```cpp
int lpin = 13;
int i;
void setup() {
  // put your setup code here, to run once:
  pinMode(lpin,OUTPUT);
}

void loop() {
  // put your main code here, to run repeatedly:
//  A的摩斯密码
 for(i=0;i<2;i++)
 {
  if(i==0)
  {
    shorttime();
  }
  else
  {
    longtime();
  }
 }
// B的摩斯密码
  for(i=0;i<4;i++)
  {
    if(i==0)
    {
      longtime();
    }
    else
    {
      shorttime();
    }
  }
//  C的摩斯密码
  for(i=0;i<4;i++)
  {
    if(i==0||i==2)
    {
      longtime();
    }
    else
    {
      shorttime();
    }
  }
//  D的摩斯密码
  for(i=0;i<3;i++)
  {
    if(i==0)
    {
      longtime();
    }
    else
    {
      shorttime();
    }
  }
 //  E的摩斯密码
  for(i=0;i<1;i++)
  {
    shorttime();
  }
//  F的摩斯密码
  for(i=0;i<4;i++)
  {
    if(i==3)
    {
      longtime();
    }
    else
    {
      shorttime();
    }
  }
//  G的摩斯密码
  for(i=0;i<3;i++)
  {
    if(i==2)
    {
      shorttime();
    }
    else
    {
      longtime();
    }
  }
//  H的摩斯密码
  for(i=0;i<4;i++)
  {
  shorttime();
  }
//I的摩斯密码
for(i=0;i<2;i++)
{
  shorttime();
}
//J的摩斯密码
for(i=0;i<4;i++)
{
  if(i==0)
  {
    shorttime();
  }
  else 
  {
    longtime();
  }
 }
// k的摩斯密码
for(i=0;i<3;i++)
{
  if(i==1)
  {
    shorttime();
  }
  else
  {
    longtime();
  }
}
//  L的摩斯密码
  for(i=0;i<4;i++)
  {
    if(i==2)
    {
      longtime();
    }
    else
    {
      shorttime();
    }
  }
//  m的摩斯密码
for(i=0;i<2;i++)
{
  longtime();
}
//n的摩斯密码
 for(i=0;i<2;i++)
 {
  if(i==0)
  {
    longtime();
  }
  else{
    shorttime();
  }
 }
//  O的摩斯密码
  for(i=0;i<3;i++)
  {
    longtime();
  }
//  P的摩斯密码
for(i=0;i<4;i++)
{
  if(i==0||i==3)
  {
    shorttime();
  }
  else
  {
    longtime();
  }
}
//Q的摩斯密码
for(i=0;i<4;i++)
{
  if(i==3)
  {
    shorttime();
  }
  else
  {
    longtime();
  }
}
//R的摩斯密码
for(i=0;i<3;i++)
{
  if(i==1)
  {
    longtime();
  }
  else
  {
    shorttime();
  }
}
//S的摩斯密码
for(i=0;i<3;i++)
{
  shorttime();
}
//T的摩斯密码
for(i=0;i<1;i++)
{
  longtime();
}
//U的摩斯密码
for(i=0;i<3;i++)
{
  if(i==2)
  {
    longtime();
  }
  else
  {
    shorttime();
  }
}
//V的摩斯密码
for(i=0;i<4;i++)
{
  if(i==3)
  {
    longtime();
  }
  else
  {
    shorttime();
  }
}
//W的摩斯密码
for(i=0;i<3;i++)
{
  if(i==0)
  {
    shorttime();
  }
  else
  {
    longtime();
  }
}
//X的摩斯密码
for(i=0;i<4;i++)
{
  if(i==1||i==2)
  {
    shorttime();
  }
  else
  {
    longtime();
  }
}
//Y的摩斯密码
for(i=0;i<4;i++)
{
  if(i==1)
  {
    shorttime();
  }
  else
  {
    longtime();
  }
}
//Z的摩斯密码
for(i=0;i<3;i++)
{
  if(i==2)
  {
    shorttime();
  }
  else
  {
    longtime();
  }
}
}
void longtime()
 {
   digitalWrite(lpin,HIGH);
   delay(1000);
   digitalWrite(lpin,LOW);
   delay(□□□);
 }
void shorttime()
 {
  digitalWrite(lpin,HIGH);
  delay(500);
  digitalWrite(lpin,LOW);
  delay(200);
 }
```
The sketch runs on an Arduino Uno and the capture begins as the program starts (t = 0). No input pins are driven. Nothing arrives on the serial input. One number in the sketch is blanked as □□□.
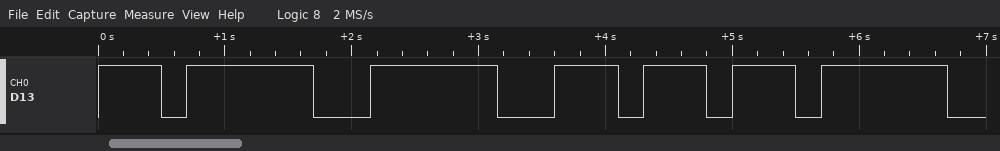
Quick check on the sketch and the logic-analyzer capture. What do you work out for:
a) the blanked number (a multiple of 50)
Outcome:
450
